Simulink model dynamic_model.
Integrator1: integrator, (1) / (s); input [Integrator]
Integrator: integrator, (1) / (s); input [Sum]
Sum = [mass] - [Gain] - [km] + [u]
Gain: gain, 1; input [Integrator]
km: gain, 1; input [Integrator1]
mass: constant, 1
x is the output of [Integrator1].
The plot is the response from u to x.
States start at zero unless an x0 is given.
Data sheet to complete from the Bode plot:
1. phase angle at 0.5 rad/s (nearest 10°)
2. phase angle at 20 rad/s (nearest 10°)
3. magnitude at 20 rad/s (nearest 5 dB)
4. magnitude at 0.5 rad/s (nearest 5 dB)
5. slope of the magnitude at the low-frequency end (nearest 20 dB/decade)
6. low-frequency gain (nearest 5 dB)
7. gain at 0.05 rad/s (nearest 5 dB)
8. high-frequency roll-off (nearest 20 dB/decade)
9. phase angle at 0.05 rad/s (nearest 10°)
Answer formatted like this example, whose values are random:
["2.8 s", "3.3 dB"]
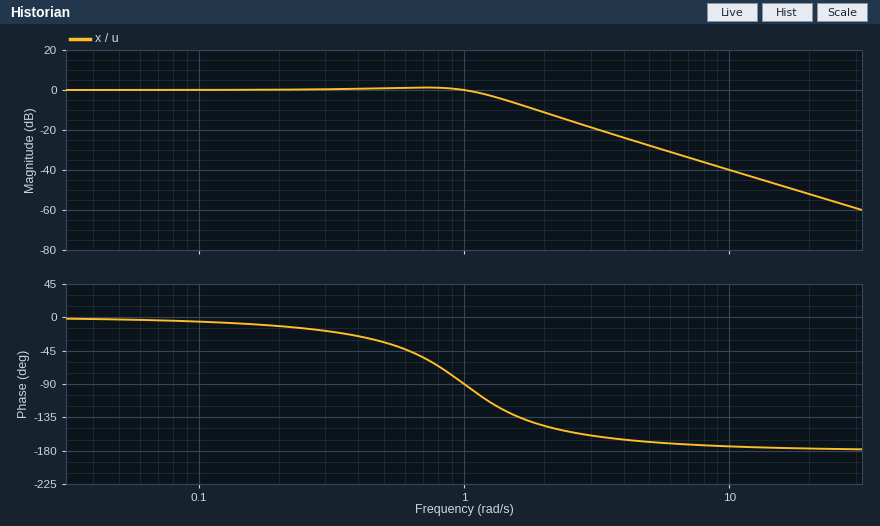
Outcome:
["-30°", "-180°", "-50 dB", "0 dB", "0 dB/decade", "0 dB", "0 dB", "-40 dB/decade", "0°"]
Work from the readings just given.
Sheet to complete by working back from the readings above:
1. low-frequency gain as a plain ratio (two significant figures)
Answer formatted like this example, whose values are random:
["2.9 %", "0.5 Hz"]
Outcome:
["1.0"]
